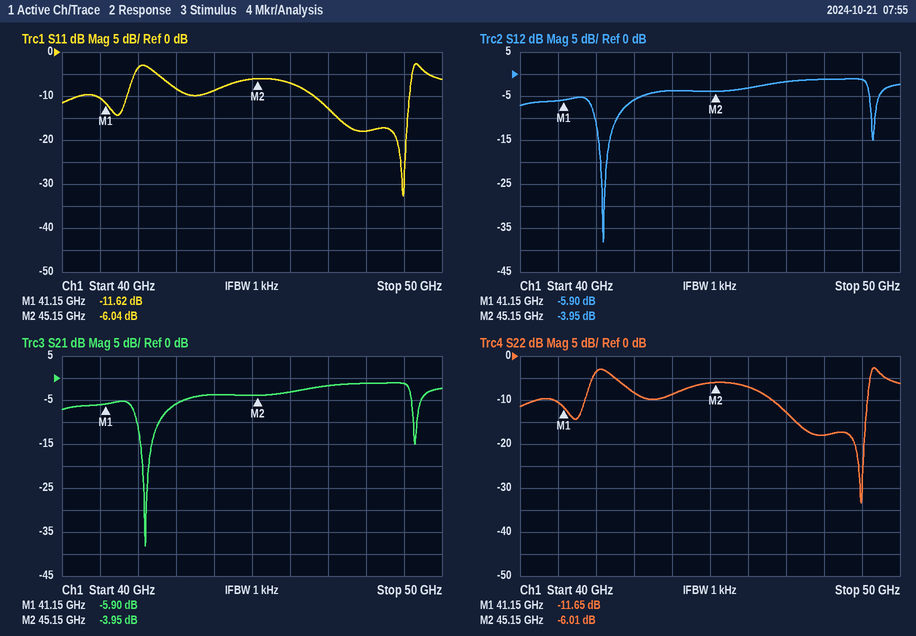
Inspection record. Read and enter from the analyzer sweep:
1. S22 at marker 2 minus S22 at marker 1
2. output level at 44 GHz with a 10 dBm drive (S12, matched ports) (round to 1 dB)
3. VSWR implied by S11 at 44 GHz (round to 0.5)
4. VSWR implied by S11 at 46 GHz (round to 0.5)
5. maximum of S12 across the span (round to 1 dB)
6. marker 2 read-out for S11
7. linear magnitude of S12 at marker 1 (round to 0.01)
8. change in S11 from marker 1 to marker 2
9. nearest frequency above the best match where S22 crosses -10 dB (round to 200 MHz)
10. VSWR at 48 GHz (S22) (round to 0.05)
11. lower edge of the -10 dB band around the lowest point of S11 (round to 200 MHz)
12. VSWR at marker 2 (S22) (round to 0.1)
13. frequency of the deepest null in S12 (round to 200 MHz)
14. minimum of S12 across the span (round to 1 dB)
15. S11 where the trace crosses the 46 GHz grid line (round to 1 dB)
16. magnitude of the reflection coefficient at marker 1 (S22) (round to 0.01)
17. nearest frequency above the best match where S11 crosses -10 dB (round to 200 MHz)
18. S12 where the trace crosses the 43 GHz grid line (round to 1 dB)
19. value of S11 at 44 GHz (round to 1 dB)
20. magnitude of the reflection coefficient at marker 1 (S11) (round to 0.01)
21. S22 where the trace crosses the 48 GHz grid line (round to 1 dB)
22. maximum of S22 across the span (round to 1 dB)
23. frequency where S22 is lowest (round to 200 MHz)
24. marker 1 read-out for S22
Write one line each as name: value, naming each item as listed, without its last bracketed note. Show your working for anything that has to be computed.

S22 at marker 2 minus S22 at marker 1: -6.01 − (-11.65) = 5.64 dB
output level at 44 GHz with a 10 dBm drive (S12, matched ports): 10 dBm + (-4 dB) = 6 dBm
VSWR implied by S11 at 44 GHz: |Γ| = 10^(-9/20) = 0.3548; VSWR = (1 + 0.3548)/(1 − 0.3548) ≈ 2.10, so 2.0 to the nearest 0.5
VSWR implied by S11 at 46 GHz: |Γ| = 10^(-7/20) = 0.4467; VSWR = (1 + 0.4467)/(1 − 0.4467) ≈ 2.61, so 2.5 to the nearest 0.5
maximum of S12 across the span: -1 dB
marker 2 read-out for S11: -6.04 dB
linear magnitude of S12 at marker 1: 10^(-5.9/20) ≈ 0.51
change in S11 from marker 1 to marker 2: -6.04 − (-11.62) = 5.58 dB
nearest frequency above the best match where S22 crosses -10 dB: 49.2 GHz
VSWR at 48 GHz (S22): |Γ| = 10^(-18/20) = 0.1259; VSWR = (1 + 0.1259)/(1 − 0.1259) ≈ 1.29, so 1.30 to the nearest 0.05
lower edge of the -10 dB band around the lowest point of S11: 46.6 GHz
VSWR at marker 2 (S22): (1 + 0.5006)/(1 − 0.5006) ≈ 3.0
frequency of the deepest null in S12: 42.2 GHz
minimum of S12 across the span: -38 dB
S11 where the trace crosses the 46 GHz grid line: -7 dB
magnitude of the reflection coefficient at marker 1 (S22): 10^(-11.65/20) ≈ 0.26
nearest frequency above the best match where S11 crosses -10 dB: 49.2 GHz
S12 where the trace crosses the 43 GHz grid line: -6 dB
value of S11 at 44 GHz: -9 dB
magnitude of the reflection coefficient at marker 1 (S11): 10^(-11.62/20) ≈ 0.26
S22 where the trace crosses the 48 GHz grid line: -18 dB
maximum of S22 across the span: -3 dB
frequency where S22 is lowest: 49.0 GHz
marker 1 read-out for S22: -11.65 dB
